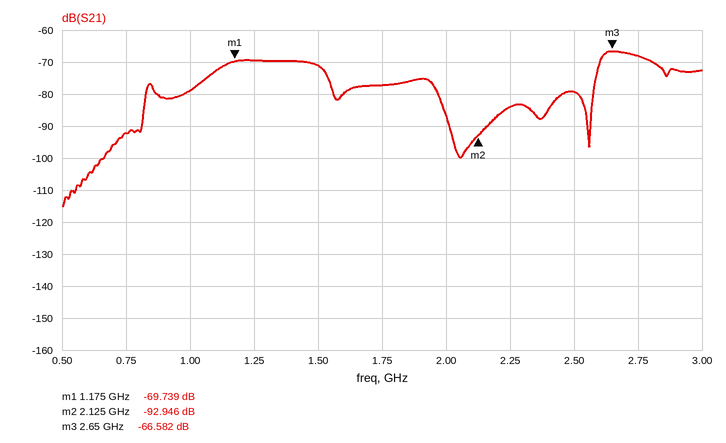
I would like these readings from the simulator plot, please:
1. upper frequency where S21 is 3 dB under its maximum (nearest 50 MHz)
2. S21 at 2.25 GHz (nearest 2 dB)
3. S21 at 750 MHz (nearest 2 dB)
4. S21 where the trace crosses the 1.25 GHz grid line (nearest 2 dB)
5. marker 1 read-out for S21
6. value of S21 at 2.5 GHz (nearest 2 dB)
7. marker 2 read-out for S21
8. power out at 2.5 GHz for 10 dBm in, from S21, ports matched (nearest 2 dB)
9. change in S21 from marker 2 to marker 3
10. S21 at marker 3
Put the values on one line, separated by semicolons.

2.80 GHz; -84 dB; -92 dB; -70 dB; -69.739 dB; -80 dB; -92.946 dB; -70 dBm; 26.364 dB; -66.582 dB
